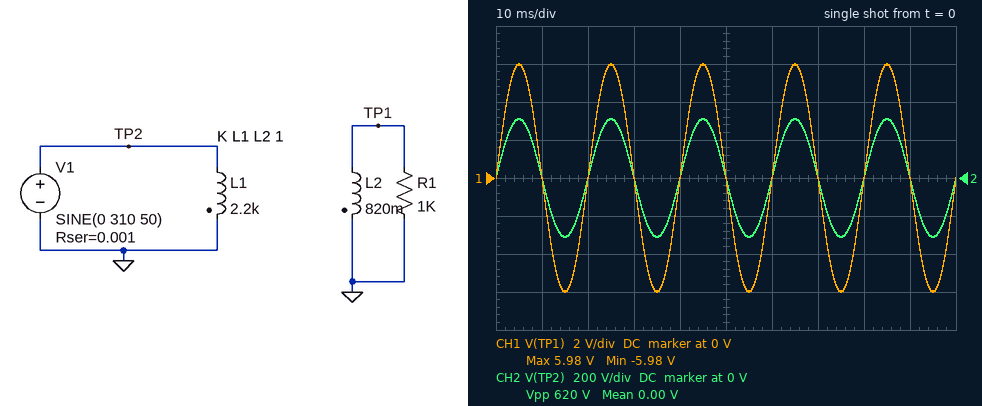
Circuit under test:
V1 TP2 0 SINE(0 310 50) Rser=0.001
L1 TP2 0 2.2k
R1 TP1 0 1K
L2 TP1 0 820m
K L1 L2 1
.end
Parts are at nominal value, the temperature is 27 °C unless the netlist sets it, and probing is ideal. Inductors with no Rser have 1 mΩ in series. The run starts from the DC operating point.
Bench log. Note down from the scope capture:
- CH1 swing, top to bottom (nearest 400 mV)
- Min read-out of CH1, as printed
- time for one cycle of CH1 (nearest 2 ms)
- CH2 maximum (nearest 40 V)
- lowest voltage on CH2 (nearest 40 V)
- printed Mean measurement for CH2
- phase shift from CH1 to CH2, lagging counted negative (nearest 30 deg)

12.0 V
-5.98 V
20 ms
320 V
-320 V
0.00 V
0 deg
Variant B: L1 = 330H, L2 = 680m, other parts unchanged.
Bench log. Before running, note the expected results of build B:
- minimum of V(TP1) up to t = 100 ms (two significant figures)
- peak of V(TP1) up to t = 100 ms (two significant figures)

-14 V
14 V
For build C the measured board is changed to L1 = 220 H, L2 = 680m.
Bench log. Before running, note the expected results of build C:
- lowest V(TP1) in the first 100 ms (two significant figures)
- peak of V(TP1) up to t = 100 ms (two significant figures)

-17 V
17 V
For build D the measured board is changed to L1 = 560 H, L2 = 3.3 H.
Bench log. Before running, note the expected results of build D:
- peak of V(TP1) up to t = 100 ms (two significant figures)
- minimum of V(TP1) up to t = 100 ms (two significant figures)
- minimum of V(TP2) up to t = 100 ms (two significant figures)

24 V
-24 V
-310 V
